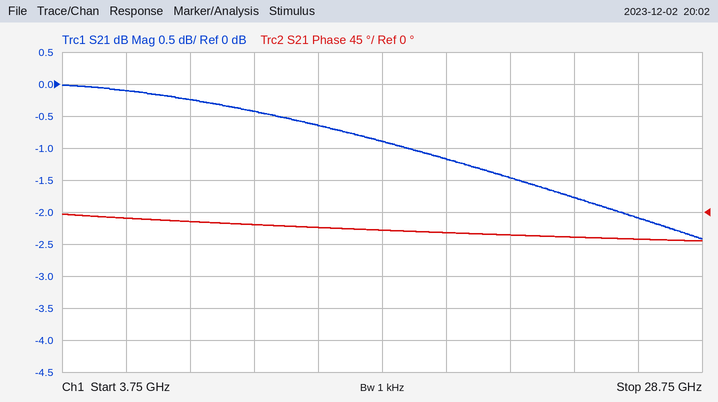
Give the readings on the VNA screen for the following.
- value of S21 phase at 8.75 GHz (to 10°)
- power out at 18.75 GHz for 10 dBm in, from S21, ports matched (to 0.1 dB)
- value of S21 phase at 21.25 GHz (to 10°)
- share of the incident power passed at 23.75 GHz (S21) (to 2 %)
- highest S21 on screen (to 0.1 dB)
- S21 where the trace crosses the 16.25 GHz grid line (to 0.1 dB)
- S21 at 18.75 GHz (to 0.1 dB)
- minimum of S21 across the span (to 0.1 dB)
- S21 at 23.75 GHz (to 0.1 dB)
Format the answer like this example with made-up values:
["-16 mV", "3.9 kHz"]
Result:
["-10°", "8.8 dBm", "-30°", "66 %", "0.0 dB", "-0.9 dB", "-1.2 dB", "-2.4 dB", "-1.8 dB"]
